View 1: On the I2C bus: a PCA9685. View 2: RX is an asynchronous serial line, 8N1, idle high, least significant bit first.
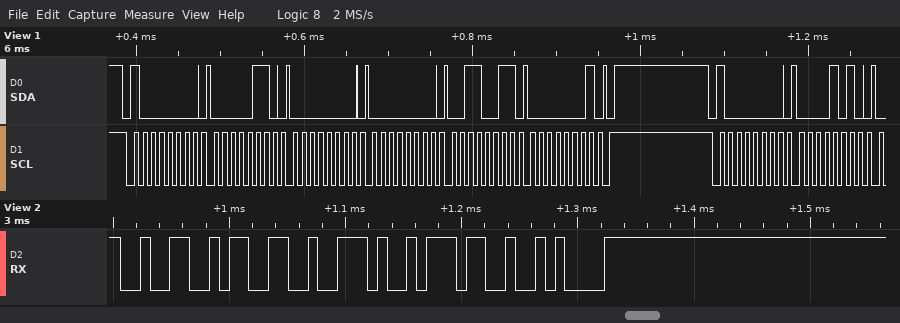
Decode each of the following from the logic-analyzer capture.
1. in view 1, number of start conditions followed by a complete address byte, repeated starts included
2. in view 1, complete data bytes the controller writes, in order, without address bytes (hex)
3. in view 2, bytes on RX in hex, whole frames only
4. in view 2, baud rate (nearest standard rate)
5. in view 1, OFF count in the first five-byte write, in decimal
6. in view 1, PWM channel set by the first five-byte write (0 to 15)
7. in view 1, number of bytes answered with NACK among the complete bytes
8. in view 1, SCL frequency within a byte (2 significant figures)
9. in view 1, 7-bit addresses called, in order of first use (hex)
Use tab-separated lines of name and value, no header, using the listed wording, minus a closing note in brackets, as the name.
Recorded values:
in view 1, number of start conditions followed by a complete address byte, repeated starts included	2
in view 1, complete data bytes the controller writes, in order, without address bytes	06 00 00 33 01 0A
in view 2, bytes on RX in hex, whole frames only	0x32 0x33 0x2E 0x37 0x0A
in view 2, baud rate	115200 baud
in view 1, OFF count in the first five-byte write, in decimal	307
in view 1, PWM channel set by the first five-byte write	0
in view 1, number of bytes answered with NACK among the complete bytes	0
in view 1, SCL frequency within a byte	100 kHz
in view 1, 7-bit addresses called, in order of first use	0x40
